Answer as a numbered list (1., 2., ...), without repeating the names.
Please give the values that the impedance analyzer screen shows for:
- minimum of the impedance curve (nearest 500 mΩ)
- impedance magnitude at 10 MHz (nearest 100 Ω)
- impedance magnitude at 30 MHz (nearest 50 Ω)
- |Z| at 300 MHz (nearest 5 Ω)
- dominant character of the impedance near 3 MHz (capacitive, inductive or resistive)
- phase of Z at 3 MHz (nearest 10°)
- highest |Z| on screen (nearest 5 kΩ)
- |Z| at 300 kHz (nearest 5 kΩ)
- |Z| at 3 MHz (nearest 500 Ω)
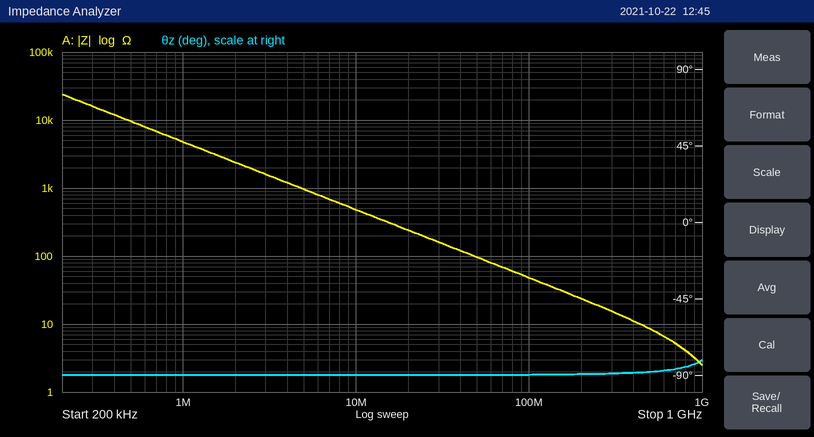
1. 2.5 Ω
2. 500 Ω
3. 150 Ω
4. 15 Ω
5. capacitive
6. -90°
7. 25 kΩ
8. 15 kΩ
9. 1.5 kΩ
